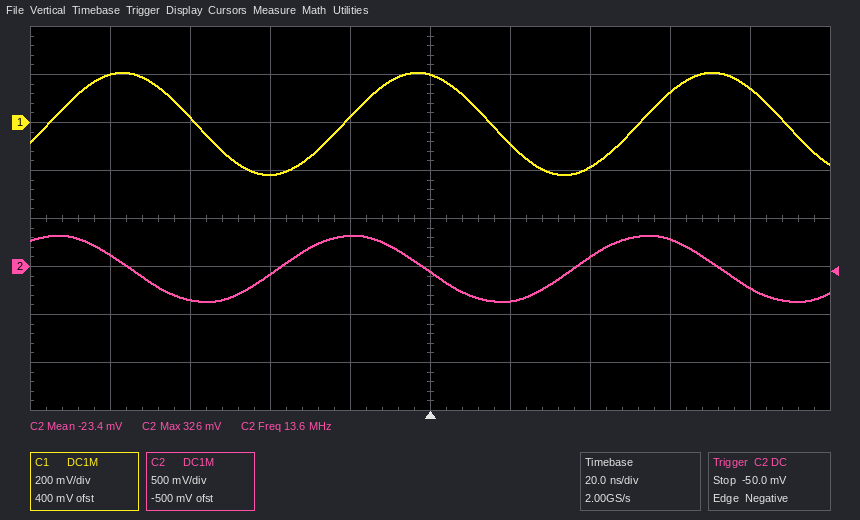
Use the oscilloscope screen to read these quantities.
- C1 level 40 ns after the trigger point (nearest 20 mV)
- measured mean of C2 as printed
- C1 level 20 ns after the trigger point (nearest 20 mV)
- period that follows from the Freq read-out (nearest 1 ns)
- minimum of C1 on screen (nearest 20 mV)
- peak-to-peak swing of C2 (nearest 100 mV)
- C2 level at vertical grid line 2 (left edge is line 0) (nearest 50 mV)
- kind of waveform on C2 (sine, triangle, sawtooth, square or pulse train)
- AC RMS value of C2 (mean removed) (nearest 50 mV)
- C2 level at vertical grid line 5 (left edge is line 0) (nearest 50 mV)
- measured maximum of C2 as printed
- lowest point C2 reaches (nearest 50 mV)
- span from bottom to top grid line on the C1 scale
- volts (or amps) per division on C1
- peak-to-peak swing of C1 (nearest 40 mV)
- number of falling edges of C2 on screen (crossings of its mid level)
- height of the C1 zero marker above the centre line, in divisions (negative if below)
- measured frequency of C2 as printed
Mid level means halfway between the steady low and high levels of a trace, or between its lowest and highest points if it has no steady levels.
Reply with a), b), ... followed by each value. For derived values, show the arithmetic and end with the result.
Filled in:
a) -180 mV
b) -23.4 mV
c) -80 mV
d) 1 / 13.6 MHz ≈ 74 ns
e) -220 mV
f) 700 mV
g) -350 mV
h) sine
i) 700 mV / (2√2) ≈ 247 mV, so 250 mV to the nearest 50 mV
j) -50 mV
k) 326 mV
l) -350 mV
m) 1.6 V
n) 200 mV
o) 440 mV
p) 3
q) +2.0 div
r) 13.6 MHz
